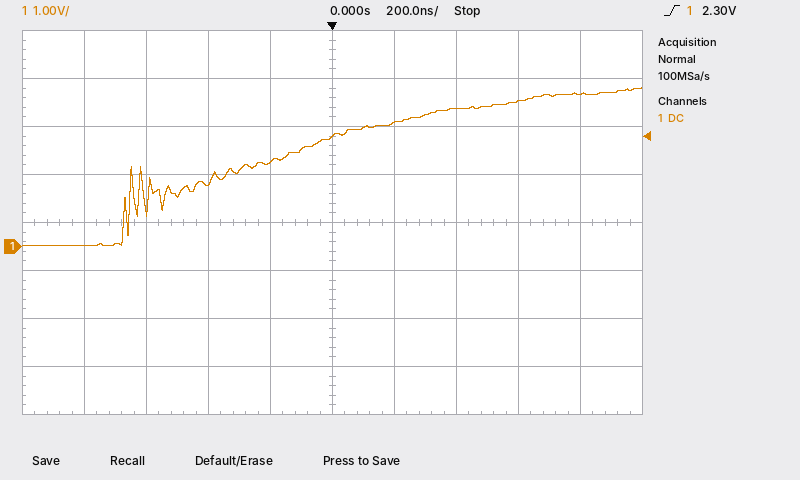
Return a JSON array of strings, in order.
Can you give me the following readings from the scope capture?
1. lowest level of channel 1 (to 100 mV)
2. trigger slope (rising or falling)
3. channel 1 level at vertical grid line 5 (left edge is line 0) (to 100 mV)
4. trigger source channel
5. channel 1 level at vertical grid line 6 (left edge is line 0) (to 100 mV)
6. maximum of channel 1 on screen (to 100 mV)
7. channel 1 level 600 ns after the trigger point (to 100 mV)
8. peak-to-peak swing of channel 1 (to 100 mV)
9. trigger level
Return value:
["0.0 V", "rising", "2.3 V", "channel 1", "2.6 V", "3.3 V", "3.0 V", "3.3 V", "2.30 V"]
